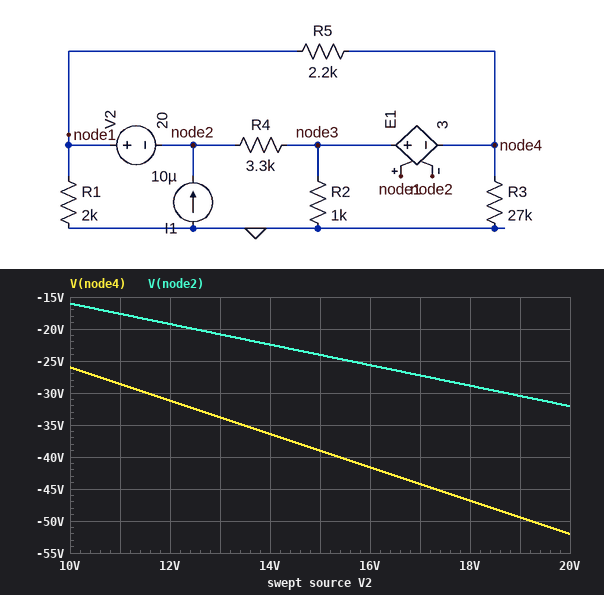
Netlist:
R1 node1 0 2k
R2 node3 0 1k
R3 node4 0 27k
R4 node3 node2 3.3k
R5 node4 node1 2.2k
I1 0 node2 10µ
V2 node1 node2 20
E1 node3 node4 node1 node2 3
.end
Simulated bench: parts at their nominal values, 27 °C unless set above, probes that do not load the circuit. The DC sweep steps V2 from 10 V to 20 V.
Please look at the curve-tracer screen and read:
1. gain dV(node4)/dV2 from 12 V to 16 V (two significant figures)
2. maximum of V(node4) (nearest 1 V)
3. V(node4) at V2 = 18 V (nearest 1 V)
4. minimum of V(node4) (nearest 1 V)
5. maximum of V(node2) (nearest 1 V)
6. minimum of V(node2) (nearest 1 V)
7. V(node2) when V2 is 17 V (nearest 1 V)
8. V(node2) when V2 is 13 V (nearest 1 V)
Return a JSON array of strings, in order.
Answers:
["-2.6 V/V", "-26 V", "-47 V", "-52 V", "-16 V", "-32 V", "-27 V", "-21 V"]
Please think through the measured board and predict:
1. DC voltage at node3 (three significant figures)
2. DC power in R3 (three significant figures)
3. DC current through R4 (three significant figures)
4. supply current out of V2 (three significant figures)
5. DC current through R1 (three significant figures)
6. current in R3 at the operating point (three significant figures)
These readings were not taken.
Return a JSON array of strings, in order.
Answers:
["7.97 V", "100 mW", "12.1 mA", "12.1 mA", "6.03 mA", "1.93 mA"]
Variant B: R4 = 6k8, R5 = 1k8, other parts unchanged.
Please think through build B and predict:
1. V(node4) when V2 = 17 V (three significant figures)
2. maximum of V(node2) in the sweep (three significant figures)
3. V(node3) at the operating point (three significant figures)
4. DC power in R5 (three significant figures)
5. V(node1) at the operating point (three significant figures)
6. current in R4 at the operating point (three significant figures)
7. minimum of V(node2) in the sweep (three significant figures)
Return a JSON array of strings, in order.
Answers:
["-41.5 V", "-19.4 V", "11.2 V", "503 mW", "-18.7 V", "7.34 mA", "-38.7 V"]
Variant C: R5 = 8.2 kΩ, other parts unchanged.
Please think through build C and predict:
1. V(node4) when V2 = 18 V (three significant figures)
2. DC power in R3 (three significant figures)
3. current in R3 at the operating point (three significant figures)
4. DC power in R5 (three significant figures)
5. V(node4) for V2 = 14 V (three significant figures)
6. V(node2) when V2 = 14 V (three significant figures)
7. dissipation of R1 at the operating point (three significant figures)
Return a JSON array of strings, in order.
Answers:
["-51.9 V", "123 mW", "2.14 mA", "402 mW", "-40.4 V", "-14.2 V", "43.1 µW"]
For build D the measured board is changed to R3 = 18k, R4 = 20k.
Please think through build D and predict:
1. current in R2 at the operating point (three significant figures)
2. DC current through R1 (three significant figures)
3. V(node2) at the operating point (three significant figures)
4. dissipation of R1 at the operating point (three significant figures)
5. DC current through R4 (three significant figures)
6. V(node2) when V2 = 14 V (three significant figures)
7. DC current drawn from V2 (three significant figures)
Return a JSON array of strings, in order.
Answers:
["12.6 mA", "9.92 mA", "-39.8 V", "197 mW", "2.62 mA", "-27.9 V", "2.63 mA"]
